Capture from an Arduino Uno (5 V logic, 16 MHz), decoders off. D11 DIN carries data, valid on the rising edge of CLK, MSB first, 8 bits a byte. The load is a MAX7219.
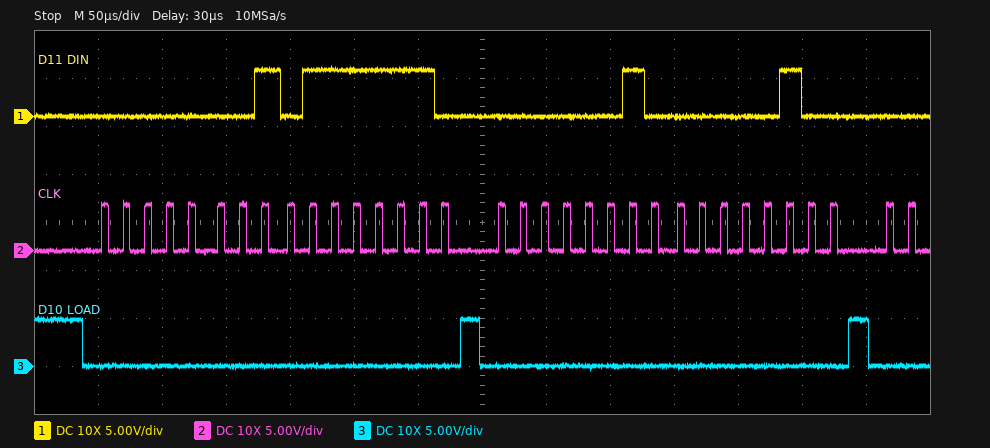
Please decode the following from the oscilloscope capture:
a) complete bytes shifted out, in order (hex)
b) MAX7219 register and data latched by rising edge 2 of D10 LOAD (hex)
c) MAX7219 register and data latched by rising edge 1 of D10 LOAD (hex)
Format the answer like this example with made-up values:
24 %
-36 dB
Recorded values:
0x01 0x7E 0x02 0x04
register 0x2, data 0x04
register 0x1, data 0x7E
